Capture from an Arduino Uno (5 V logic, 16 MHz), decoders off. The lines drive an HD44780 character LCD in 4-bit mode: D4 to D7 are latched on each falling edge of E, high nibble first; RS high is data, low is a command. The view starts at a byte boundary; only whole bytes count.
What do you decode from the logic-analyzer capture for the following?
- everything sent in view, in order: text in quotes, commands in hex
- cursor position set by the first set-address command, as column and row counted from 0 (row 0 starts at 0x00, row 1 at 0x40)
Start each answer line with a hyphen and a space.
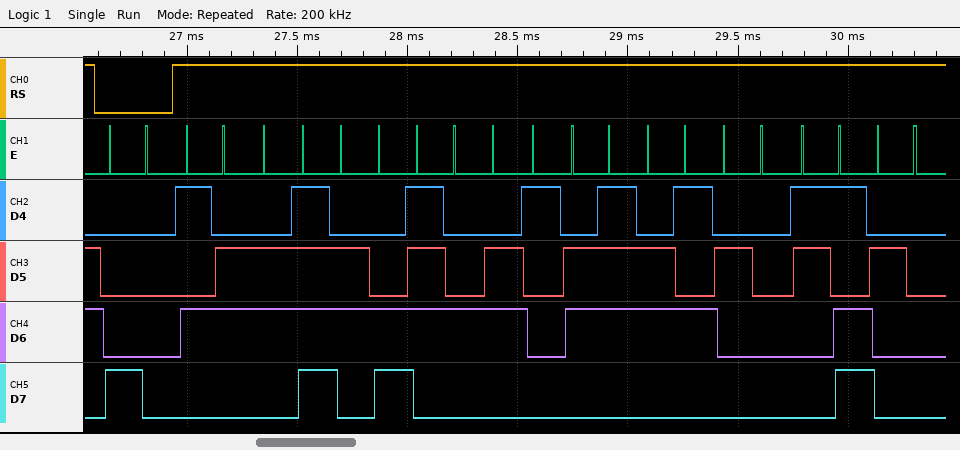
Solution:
- 0x80 "Voltage = "
- column 0, row 0
